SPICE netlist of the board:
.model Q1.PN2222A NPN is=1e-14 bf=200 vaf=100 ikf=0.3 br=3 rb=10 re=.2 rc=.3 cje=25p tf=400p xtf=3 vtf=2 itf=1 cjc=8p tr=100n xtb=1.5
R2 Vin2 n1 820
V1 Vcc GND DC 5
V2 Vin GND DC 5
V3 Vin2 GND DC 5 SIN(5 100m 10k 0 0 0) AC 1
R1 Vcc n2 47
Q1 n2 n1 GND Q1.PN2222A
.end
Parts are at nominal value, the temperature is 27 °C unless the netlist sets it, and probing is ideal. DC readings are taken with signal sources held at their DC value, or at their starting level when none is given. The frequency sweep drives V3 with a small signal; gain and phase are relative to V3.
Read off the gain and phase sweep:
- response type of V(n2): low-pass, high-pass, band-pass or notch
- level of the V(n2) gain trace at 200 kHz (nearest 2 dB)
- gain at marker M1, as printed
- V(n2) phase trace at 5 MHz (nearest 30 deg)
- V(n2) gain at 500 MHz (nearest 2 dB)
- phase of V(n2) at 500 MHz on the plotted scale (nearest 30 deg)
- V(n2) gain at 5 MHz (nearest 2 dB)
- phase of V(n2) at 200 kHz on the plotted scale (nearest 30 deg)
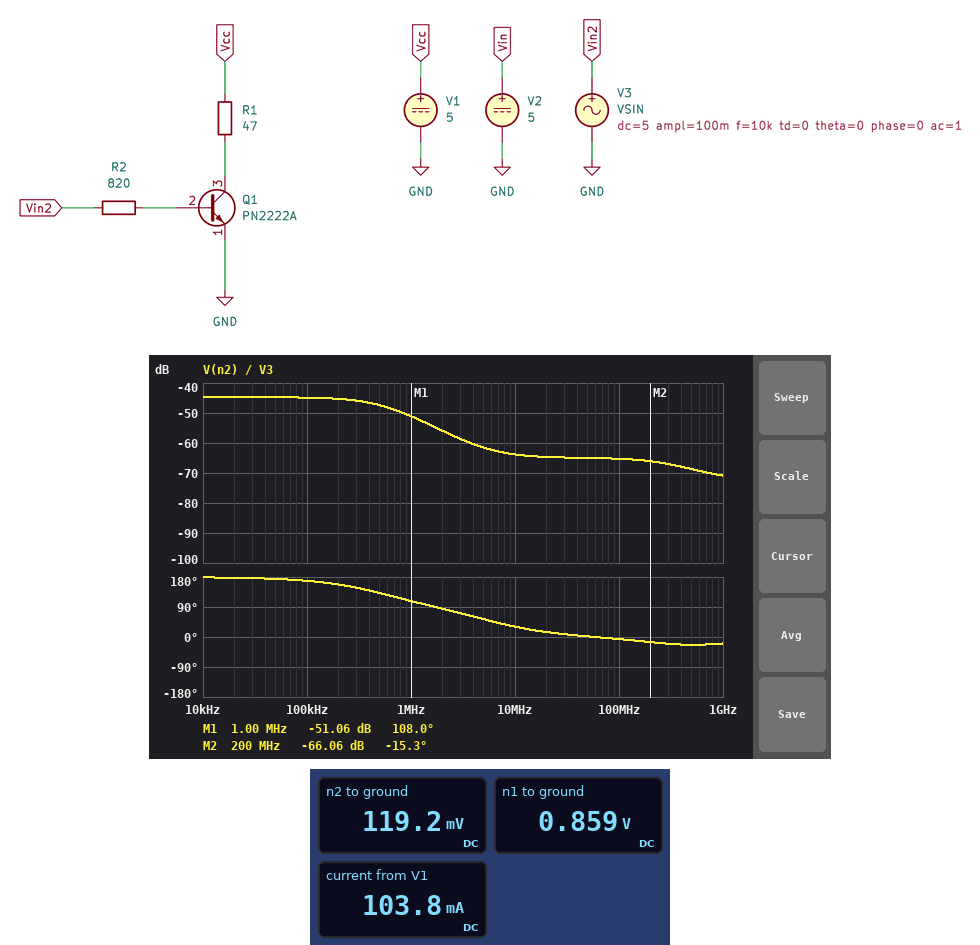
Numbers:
low-pass
-46 dB
-51.06 dB
60 deg
-68 dB
-30 deg
-62 dB
150 deg
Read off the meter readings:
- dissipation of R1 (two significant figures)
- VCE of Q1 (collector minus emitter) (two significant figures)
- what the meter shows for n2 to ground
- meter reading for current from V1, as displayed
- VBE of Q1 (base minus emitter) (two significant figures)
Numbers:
510 mW
120 mV
119.2 mV
103.8 mA
860 mV
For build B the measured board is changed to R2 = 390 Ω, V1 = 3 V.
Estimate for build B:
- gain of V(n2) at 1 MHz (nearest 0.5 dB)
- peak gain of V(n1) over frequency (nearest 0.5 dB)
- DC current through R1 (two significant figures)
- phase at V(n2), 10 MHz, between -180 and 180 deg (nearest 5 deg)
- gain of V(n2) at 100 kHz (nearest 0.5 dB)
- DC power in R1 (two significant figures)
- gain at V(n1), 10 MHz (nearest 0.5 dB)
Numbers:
-54.5 dB
-31.0 dB
62 mA
10 deg
-50.0 dB
180 mW
-31.5 dB
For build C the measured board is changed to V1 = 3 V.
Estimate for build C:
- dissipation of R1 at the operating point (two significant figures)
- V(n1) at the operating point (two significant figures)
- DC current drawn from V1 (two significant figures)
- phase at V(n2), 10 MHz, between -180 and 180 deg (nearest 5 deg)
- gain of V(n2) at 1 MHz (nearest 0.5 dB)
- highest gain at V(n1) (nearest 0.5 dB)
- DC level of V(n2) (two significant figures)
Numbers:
180 mW
840 mV
62 mA
20 deg
-52.5 dB
-37.0 dB
83 mV
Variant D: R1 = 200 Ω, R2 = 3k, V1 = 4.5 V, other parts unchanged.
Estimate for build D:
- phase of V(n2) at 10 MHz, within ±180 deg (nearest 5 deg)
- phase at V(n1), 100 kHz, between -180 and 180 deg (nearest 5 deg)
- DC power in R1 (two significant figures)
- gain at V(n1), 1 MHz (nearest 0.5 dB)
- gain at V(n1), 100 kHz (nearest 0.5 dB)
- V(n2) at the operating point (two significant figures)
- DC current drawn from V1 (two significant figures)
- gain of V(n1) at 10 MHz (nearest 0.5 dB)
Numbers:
35 deg
0 deg
98 mW
-48.0 dB
-46.5 dB
64 mV
22 mA
-48.5 dB
